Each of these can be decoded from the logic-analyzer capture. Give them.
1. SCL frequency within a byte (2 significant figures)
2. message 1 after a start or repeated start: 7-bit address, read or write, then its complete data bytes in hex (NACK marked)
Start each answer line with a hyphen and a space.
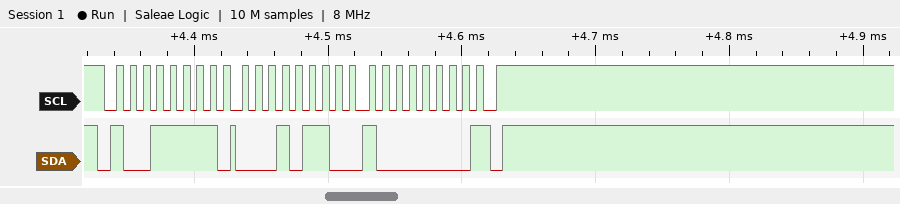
- 100 kHz
- 0x4F read: 16 80 NACK
